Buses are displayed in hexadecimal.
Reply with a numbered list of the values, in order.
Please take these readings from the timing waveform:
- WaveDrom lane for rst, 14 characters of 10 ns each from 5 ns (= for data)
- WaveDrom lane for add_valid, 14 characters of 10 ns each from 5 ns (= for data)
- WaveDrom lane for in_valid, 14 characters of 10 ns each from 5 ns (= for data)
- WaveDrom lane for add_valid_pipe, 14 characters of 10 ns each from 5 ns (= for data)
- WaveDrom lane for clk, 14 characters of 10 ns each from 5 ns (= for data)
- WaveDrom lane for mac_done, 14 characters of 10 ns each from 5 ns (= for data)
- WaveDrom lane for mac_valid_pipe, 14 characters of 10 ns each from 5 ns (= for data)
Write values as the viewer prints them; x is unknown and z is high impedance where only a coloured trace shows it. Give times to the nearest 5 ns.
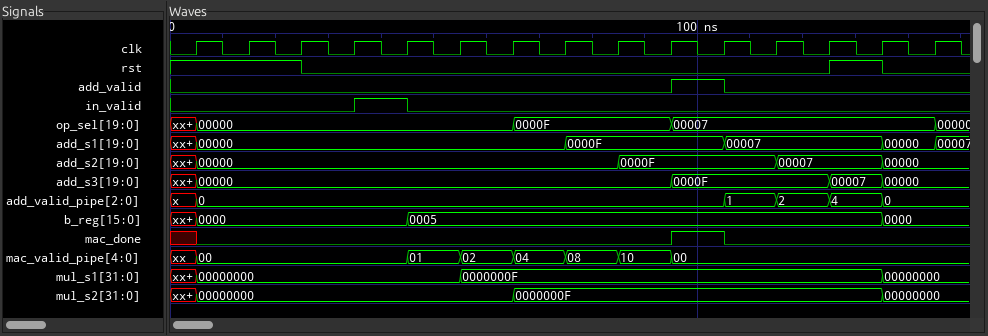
1. {name: 'rst', wave: '1.0.........10'}
2. {name: 'add_valid', wave: '0........10...'}
3. {name: 'in_valid', wave: '0..10.........'}
4. {name: 'add_valid_pipe', wave: '=.........====', data: '0 1 2 4 0'}
5. {name: 'clk', wave: 'p.............'}
6. {name: 'mac_done', wave: '0........10...'}
7. {name: 'mac_valid_pipe', wave: '=...======....', data: '00 01 02 04 08 10 00'}
